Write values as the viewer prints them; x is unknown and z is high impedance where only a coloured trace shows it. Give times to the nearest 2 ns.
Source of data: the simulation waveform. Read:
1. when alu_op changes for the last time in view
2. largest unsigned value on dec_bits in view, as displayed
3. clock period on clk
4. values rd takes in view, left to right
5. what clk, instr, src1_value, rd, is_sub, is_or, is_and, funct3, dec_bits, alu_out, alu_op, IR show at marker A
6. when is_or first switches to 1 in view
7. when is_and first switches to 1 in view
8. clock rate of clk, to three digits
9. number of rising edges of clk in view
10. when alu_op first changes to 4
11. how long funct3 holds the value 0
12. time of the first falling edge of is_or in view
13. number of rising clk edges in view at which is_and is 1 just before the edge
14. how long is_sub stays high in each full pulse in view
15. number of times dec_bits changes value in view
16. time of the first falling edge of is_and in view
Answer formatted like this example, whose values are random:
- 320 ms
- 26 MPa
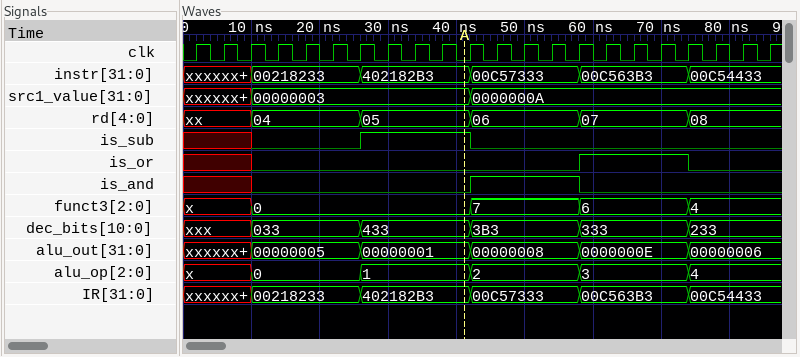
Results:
- 74 ns
- 433
- 4 ns
- xx, 04, 05, 06, 07, 08
- clk=0, instr=402182B3, src1_value=00000003, rd=05, is_sub=1, is_or=0, is_and=0, funct3=0, dec_bits=433, alu_out=00000001, alu_op=1, IR=402182B3
- 58 ns
- 42 ns
- 250 MHz
- 22
- 74 ns
- 32 ns
- 74 ns
- 4
- 16 ns
- 5
- 58 ns
